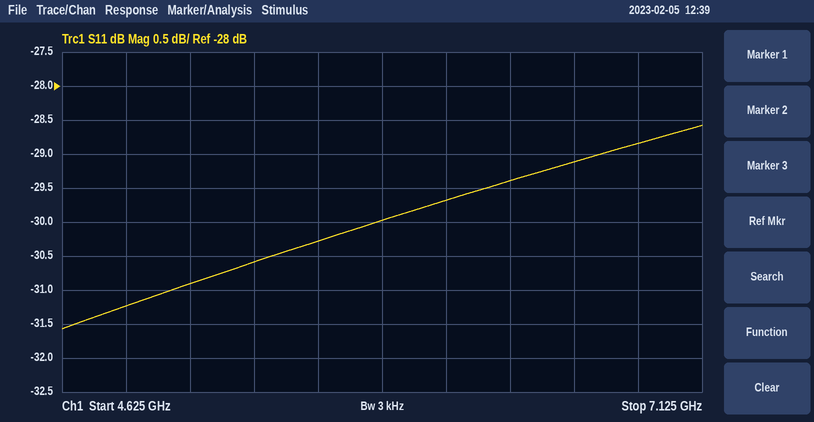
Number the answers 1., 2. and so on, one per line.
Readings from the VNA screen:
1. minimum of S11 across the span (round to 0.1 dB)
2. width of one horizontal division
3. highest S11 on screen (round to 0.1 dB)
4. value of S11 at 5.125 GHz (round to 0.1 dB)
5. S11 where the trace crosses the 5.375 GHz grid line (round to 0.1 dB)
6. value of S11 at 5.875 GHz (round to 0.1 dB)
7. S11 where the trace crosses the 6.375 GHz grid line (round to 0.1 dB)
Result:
1. -31.6 dB
2. 250 MHz
3. -28.6 dB
4. -30.9 dB
5. -30.6 dB
6. -30.0 dB
7. -29.4 dB
